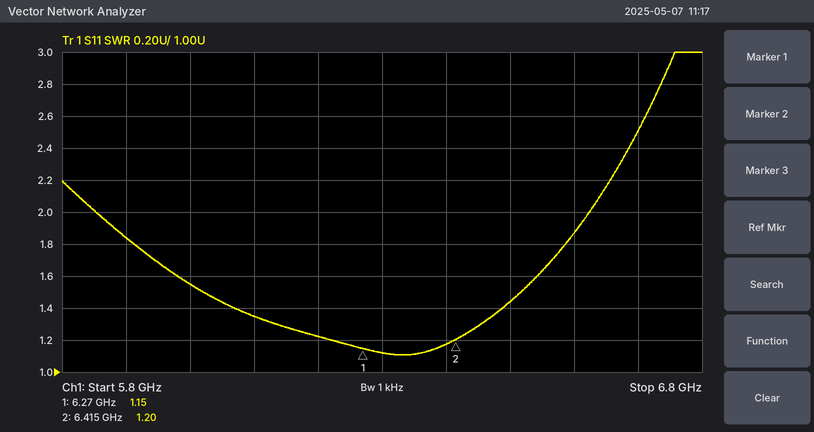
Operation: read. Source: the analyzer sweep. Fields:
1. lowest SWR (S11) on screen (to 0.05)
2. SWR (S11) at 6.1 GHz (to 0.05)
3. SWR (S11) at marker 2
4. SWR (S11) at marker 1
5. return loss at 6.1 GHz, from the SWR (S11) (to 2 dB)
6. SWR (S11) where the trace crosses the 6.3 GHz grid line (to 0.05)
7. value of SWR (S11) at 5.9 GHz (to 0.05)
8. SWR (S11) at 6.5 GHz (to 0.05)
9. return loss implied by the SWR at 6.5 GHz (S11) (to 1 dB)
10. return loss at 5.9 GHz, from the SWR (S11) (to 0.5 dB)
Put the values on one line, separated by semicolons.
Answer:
1.10; 1.35; 1.20; 1.15; 16 dB; 1.10; 1.85; 1.45; 15 dB; 10.5 dB
